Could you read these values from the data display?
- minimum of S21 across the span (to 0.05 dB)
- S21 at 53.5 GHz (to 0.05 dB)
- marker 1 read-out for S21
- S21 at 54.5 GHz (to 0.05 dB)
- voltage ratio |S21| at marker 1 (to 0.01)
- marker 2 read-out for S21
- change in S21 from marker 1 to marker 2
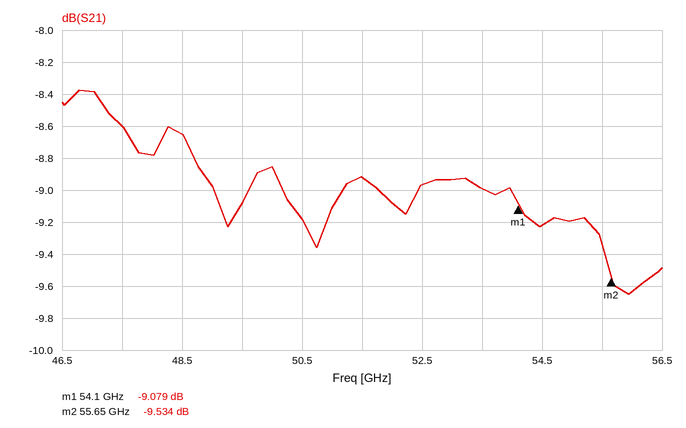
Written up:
-9.65 dB
-9.00 dB
-9.079 dB
-9.20 dB
0.35
-9.534 dB
-0.455 dB
